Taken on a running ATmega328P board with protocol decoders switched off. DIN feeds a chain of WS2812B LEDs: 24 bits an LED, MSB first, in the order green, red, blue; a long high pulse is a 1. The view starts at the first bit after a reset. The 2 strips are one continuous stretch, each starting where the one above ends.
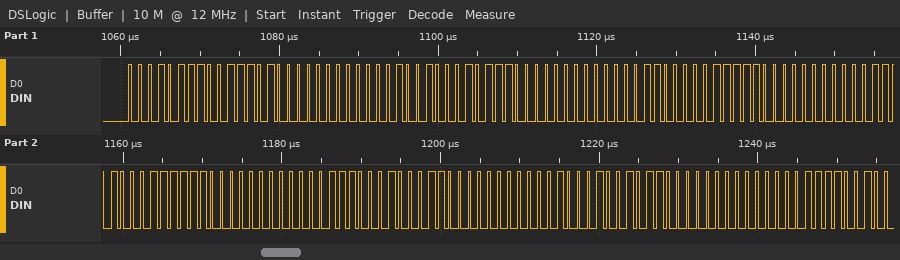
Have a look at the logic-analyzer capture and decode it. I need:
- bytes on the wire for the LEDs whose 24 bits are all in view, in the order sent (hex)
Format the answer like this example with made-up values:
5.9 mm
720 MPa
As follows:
17 3A 00 12 2E 00 0C 1F 00 1A 3F 00 0E 23 00 11 2C 00
